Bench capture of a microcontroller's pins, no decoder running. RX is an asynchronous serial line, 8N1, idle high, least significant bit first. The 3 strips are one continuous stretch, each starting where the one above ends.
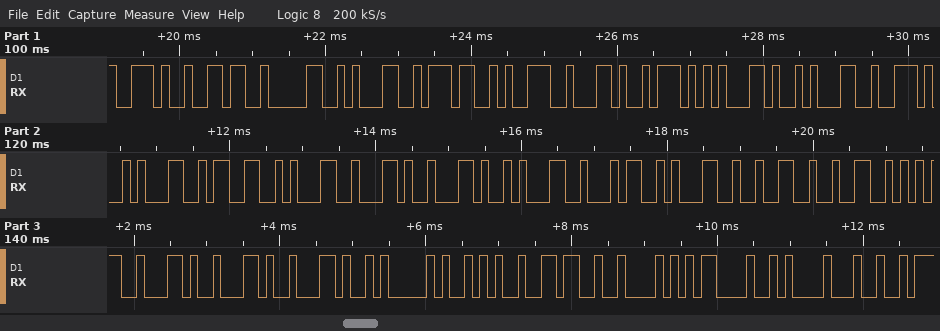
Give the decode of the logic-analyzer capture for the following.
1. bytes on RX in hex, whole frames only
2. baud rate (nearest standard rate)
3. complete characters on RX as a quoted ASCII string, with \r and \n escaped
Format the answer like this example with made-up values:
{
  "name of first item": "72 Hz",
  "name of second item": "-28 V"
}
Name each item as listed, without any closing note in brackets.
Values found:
{
  "bytes on RX in hex, whole frames only": "2E 36 30 31 37 39 2C 57 2C 31 2E 31 33 31 2C 2C 31 34 31 32 32 35 2C 2C 2C 41 2A 36 42 0D 0A 24",
  "baud rate": "9600 baud",
  "complete characters on RX as a quoted ASCII string, with \\r and \\n escaped": "\".60179,W,1.131,,141225,,,A*6B\\r\\n$\""
}
